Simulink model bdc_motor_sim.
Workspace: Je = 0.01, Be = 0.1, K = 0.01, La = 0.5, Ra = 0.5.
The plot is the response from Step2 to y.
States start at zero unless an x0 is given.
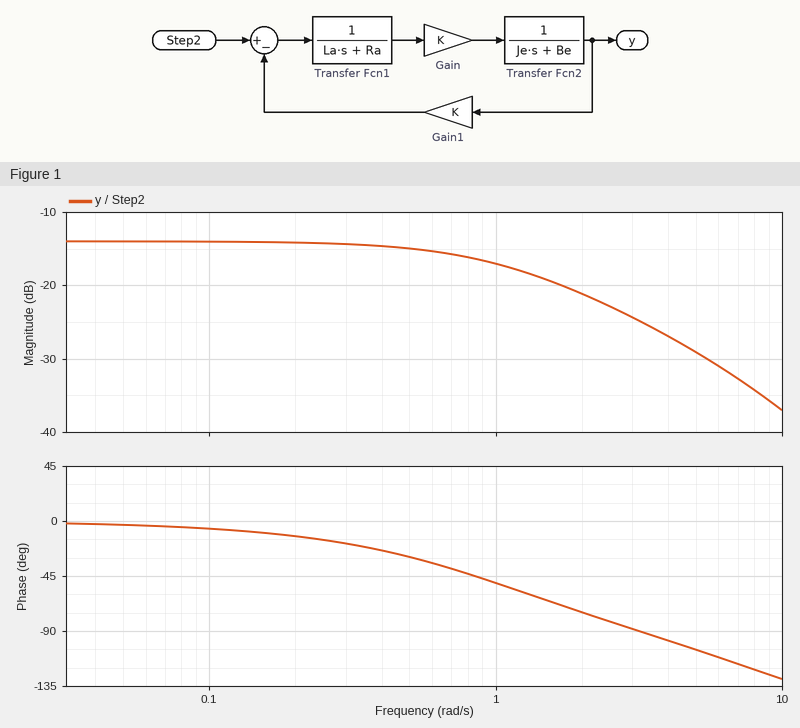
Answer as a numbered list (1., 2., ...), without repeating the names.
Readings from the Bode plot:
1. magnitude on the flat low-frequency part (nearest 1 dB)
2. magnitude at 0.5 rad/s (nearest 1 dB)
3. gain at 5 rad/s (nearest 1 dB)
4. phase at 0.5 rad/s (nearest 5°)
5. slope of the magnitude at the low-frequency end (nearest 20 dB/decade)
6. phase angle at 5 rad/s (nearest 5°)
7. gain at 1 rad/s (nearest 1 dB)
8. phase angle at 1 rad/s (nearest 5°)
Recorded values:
1. -14 dB
2. -15 dB
3. -29 dB
4. -30°
5. 0 dB/decade
6. -105°
7. -17 dB
8. -50°
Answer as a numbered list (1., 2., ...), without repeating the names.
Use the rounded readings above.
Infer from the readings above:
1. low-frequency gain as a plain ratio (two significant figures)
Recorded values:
1. 0.20
